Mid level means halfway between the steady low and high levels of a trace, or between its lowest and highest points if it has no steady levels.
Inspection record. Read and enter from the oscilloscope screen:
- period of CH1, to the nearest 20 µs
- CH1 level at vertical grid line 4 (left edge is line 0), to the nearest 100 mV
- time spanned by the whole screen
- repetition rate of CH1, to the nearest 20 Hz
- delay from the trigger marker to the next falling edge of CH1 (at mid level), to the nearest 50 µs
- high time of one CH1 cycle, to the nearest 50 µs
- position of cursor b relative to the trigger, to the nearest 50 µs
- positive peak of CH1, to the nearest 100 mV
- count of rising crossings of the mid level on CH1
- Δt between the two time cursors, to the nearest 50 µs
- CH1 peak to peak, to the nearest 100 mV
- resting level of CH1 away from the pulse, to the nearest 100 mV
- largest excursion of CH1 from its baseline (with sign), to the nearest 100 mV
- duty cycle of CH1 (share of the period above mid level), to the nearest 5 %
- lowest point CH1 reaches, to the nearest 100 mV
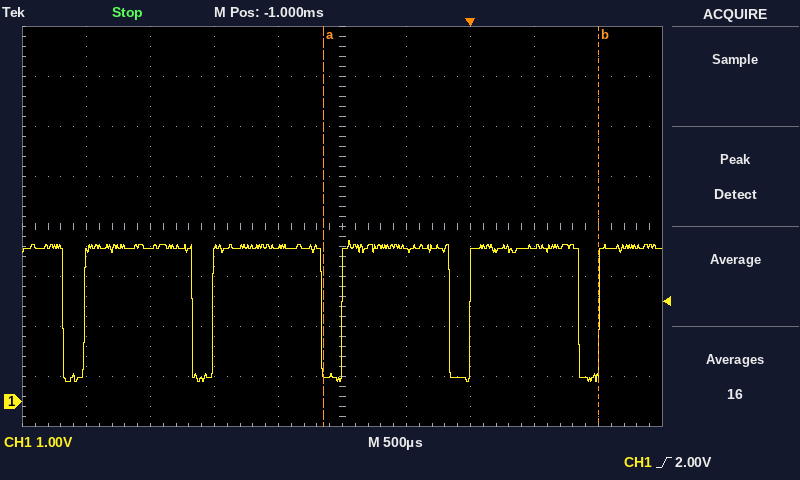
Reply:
1.00 ms
3.1 V
5 ms
1.00 kHz
850 µs
850 µs
+1.00 ms
3.2 V
5
2.15 ms
2.8 V
3.1 V
-2.7 V
85 %
400 mV
